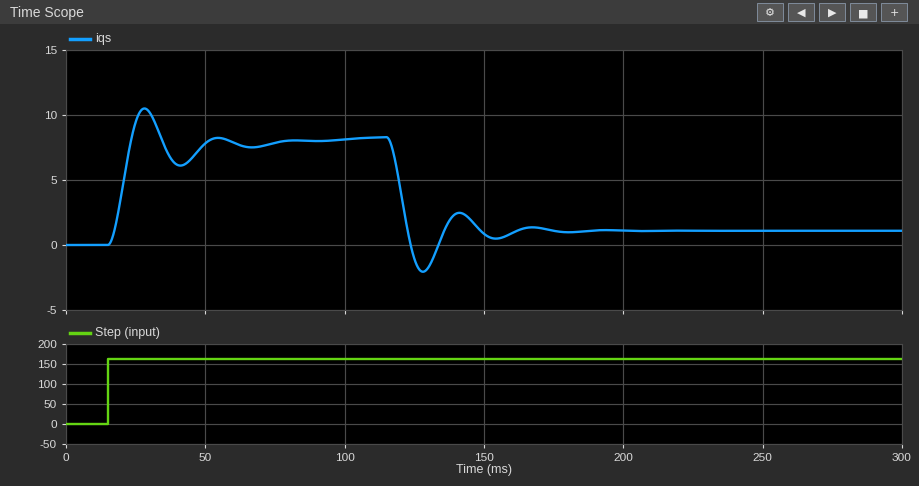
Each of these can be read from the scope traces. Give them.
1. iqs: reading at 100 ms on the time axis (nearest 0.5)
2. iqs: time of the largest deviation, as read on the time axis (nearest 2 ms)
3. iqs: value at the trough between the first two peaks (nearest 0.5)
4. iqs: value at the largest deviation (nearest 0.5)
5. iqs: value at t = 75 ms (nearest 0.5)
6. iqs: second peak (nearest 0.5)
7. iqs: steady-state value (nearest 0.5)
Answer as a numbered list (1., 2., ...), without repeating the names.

1. 8.0
2. 28 ms
3. 6.0
4. 10.5
5. 8.0
6. 8.5
7. 1.0
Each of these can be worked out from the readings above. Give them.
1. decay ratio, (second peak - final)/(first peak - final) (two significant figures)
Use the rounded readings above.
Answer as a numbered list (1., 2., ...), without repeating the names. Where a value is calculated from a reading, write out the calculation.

1. (8.5 - 1) / (10.5 - 1) = 0.79
